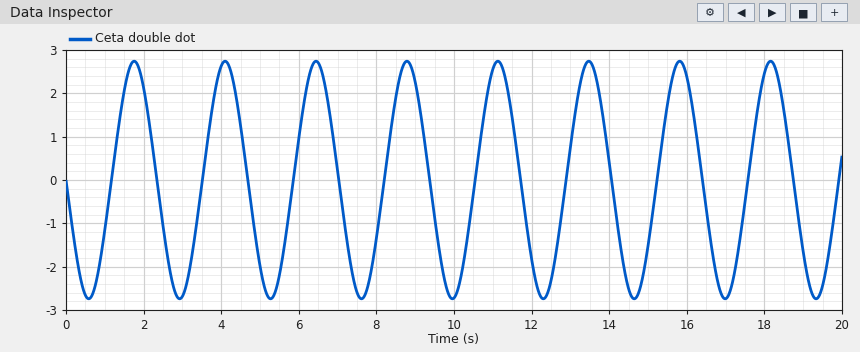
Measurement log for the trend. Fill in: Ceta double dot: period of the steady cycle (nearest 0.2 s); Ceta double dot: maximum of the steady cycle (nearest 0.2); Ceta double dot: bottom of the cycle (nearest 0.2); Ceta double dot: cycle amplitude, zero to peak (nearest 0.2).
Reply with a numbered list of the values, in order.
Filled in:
1. 2.4 s
2. 2.8
3. -2.8
4. 2.8
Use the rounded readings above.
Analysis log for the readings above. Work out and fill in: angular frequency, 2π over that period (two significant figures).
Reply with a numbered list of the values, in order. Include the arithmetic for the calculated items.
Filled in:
1. 2π / 2.4 = 2.6 rad/s
